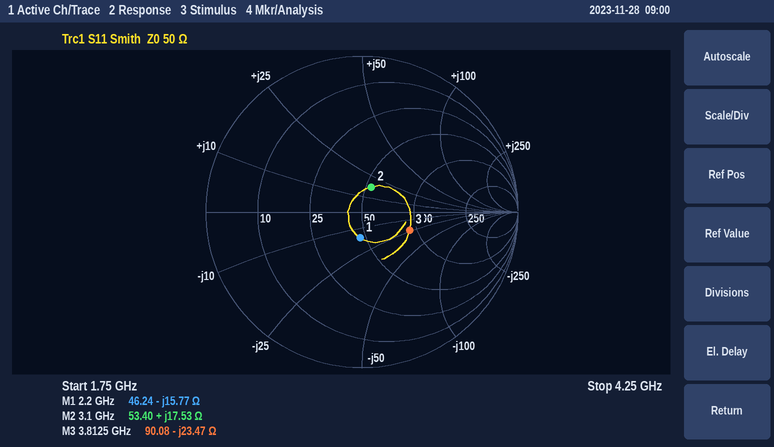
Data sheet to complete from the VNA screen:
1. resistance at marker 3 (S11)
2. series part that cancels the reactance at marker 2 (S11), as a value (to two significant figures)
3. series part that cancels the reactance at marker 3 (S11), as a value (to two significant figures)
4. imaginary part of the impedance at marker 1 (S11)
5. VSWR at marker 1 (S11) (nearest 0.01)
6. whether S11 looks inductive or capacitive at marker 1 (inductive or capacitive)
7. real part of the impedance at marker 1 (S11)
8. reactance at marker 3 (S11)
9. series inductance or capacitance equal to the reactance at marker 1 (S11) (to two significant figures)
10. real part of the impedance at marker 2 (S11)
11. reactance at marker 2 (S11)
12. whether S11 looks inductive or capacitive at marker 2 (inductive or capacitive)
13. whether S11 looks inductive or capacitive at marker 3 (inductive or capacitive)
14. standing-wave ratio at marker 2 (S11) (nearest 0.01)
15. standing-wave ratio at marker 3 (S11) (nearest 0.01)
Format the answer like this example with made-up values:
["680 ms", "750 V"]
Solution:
["90.08 Ω", "2.9 pF", "980 pH", "-15.77 Ω", "1.40", "capacitive", "46.24 Ω", "-23.47 Ω", "4.6 pF", "53.40 Ω", "+17.53 Ω", "inductive", "capacitive", "1.41", "1.97"]
